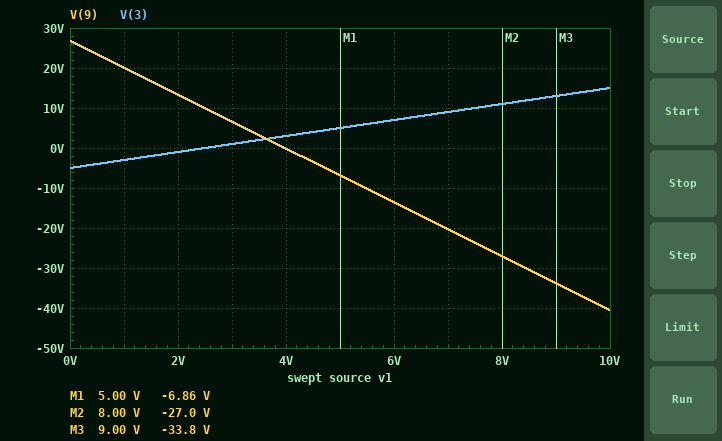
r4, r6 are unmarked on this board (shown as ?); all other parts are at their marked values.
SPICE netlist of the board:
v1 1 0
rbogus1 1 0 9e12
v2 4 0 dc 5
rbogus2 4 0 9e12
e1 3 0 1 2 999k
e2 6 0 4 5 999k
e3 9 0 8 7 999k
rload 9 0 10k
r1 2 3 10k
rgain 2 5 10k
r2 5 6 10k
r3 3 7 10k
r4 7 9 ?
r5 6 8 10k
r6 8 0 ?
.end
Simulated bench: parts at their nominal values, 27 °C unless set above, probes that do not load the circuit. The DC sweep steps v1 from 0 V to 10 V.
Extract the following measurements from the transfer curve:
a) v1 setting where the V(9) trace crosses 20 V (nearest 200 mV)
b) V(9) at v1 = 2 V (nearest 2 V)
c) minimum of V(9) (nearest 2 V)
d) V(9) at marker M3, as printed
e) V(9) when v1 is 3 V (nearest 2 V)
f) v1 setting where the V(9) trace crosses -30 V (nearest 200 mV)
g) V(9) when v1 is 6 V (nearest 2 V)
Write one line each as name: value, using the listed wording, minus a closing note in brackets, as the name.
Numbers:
v1 setting where the V(9) trace crosses 20 V: 1.0 V
V(9) at v1 = 2 V: 14 V
minimum of V(9): -40 V
V(9) at marker M3, as printed: -33.8 V
V(9) when v1 is 3 V: 6 V
v1 setting where the V(9) trace crosses -30 V: 8.4 V
V(9) when v1 is 6 V: -14 V
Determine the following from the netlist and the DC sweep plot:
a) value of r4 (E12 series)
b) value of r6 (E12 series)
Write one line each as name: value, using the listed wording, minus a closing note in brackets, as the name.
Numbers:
value of r4: 27 kΩ
value of r6: 5.6 kΩ
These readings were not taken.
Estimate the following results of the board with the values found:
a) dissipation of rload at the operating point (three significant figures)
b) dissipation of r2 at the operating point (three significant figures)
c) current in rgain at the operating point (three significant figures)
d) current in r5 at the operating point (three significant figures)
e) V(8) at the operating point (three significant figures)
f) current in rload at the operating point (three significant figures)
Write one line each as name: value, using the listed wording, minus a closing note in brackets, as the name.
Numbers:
dissipation of rload at the operating point: 71.7 mW
dissipation of r2 at the operating point: 2.50 mW
current in rgain at the operating point: 500 µA
current in r5 at the operating point: 641 µA
V(8) at the operating point: 3.59 V
current in rload at the operating point: 2.68 mA
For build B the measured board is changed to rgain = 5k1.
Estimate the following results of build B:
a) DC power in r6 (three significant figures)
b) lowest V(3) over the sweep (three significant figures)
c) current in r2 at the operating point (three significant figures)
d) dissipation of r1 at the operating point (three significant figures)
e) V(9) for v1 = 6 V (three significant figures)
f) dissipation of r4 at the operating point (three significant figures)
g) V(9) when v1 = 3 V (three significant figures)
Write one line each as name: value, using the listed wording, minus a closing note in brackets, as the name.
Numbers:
DC power in r6: 5.04 mW
lowest V(3) over the sweep: -9.80 V
current in r2 at the operating point: 980 µA
dissipation of r1 at the operating point: 9.61 mW
V(9) for v1 = 6 V: -17.5 V
dissipation of r4 at the operating point: 61.7 mW
V(9) when v1 = 3 V: 14.3 V
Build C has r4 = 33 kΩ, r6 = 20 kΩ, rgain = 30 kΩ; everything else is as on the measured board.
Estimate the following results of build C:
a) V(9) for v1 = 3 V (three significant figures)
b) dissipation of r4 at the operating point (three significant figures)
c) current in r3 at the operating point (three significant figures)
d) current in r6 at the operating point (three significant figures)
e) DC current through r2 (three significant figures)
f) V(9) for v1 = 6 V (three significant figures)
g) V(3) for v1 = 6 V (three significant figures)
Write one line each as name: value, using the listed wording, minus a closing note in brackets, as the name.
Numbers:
V(9) for v1 = 3 V: 8.54 V
dissipation of r4 at the operating point: 12.3 mW
current in r3 at the operating point: 611 µA
current in r6 at the operating point: 222 µA
DC current through r2: 167 µA
V(9) for v1 = 6 V: -7.52 V
V(3) for v1 = 6 V: 6.33 V
